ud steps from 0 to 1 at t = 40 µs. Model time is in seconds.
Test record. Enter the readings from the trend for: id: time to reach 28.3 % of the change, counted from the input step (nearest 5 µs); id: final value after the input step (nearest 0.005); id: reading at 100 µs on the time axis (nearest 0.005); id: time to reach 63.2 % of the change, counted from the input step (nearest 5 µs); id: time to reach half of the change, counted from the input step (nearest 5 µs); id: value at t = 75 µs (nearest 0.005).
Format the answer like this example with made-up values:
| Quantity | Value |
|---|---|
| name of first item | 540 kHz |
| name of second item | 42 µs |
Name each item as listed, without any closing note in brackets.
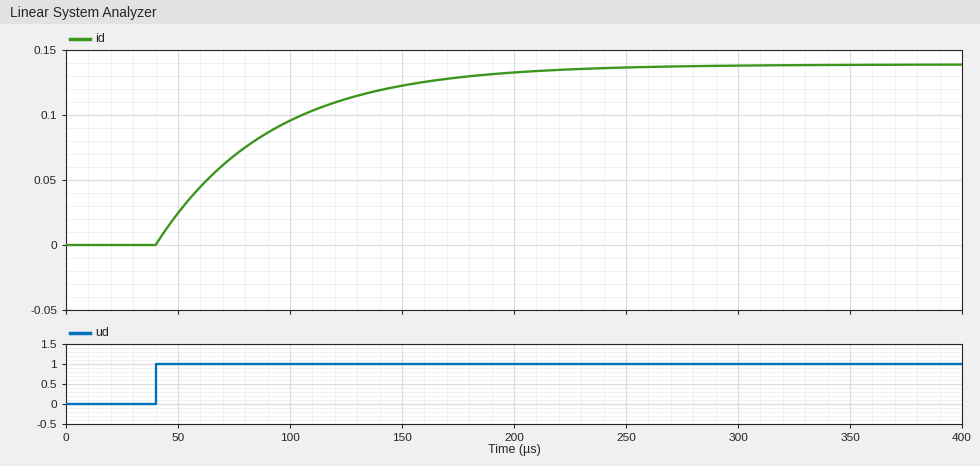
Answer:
| Quantity | Value |
|---|---|
| id: time to reach 28.3 % of the change, counted from the input step | 15 µs |
| id: final value after the input step | 0.140 |
| id: reading at 100 µs on the time axis | 0.095 |
| id: time to reach 63.2 % of the change, counted from the input step | 50 µs |
| id: time to reach half of the change, counted from the input step | 35 µs |
| id: value at t = 75 µs | 0.070 |
